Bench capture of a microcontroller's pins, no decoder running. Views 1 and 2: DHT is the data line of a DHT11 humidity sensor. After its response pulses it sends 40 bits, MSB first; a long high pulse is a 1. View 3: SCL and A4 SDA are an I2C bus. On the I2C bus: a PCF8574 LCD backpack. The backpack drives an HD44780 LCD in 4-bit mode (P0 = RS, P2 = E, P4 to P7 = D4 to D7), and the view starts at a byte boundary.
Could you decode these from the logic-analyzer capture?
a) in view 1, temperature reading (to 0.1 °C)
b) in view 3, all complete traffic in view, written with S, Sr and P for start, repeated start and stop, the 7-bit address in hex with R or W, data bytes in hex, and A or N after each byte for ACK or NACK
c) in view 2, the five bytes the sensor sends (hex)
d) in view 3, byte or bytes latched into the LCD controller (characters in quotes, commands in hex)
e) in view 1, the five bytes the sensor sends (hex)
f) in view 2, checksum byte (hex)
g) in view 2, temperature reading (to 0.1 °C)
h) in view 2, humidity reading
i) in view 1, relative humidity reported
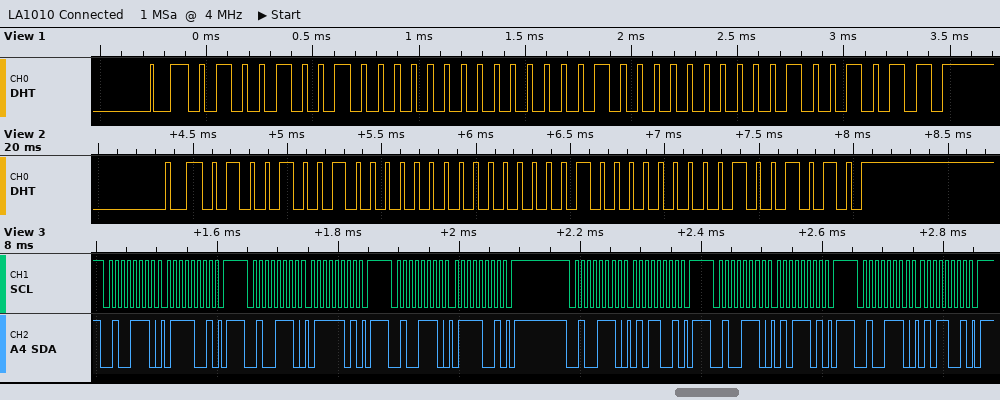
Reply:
2.0 °C
S 27W A 79 A P S 27W A 7D A P S 27W A 79 A P S 27W A 59 A P S 27W A 5D A P S 27W A 59 A P
49 00 01 00 4A
'u'
49 00 02 00 4B
0x4A
1.0 °C
73 %
73 %
